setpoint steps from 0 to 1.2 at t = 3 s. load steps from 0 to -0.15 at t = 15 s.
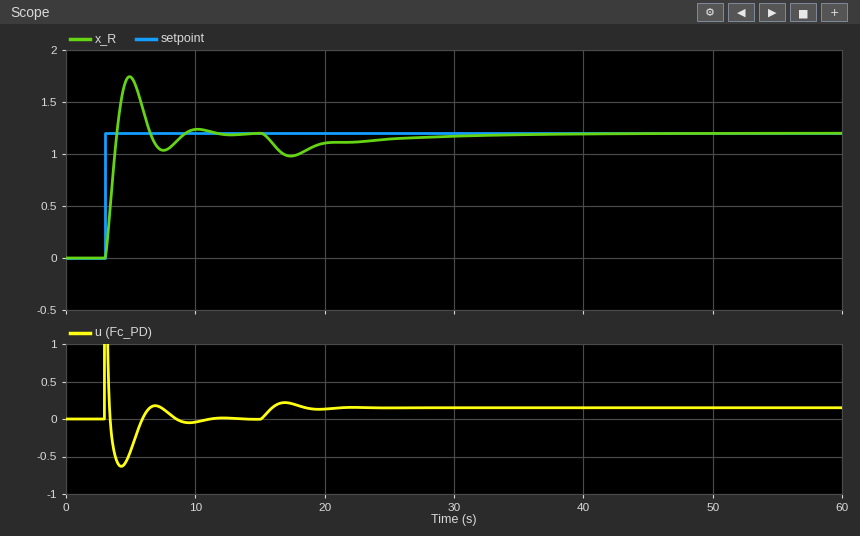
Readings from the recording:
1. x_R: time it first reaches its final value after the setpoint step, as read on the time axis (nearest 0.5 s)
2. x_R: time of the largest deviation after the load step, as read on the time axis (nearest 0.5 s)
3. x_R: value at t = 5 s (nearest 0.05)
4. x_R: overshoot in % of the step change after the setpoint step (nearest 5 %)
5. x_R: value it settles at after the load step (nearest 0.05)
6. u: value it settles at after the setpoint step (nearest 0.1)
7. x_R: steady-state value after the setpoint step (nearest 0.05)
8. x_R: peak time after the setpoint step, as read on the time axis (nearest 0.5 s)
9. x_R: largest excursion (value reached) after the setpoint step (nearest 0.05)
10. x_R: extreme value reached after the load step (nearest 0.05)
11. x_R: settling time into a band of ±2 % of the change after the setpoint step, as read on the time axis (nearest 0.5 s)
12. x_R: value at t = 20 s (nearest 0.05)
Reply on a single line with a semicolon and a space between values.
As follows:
4.0 s; 17.5 s; 1.75; 45 %; 1.20; 0.0; 1.20; 5.0 s; 1.75; 1.00; 11.0 s; 1.10
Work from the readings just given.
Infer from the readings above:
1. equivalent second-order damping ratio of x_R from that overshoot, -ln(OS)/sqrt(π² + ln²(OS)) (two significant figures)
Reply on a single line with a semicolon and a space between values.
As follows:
0.25
